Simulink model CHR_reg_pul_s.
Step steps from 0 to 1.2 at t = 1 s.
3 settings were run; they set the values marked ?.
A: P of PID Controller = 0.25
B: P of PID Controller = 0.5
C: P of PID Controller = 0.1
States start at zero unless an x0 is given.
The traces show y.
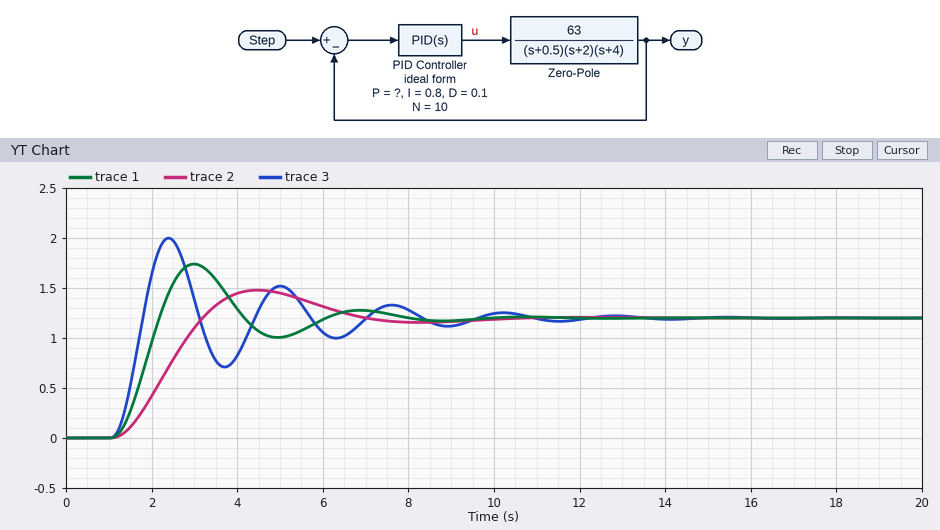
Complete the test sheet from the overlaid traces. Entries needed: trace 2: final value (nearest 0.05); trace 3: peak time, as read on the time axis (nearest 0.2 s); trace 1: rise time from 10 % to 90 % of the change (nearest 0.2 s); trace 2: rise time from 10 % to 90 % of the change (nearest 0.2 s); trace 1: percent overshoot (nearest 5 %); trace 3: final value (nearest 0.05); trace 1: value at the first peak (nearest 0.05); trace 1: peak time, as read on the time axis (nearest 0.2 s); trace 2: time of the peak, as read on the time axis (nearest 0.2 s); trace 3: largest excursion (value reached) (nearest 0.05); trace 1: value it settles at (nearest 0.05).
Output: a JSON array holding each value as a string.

["1.20", "2.4 s", "0.8 s", "1.4 s", "45 %", "1.20", "1.75", "3.0 s", "4.4 s", "2.00", "1.20"]
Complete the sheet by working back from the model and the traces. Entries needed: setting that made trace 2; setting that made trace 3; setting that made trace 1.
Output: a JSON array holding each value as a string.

["C", "B", "A"]
